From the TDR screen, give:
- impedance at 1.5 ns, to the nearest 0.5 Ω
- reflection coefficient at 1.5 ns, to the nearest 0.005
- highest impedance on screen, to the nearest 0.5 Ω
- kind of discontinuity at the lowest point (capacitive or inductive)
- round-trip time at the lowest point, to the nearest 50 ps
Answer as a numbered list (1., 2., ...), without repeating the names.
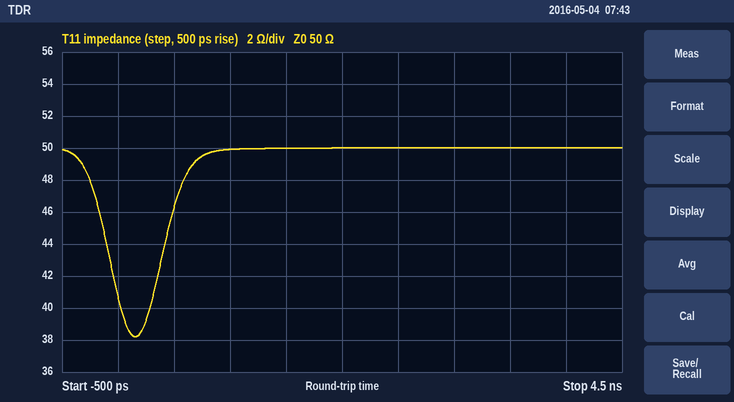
1. 50.0 Ω
2. 0.000
3. 50.0 Ω
4. capacitive
5. 150 ps
